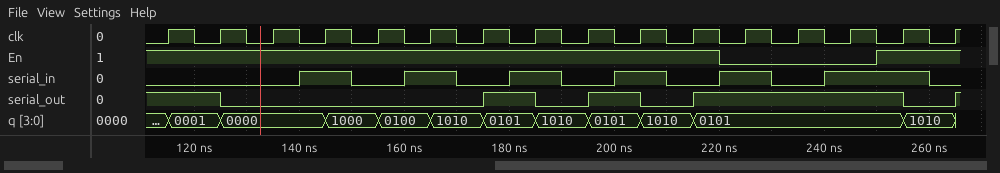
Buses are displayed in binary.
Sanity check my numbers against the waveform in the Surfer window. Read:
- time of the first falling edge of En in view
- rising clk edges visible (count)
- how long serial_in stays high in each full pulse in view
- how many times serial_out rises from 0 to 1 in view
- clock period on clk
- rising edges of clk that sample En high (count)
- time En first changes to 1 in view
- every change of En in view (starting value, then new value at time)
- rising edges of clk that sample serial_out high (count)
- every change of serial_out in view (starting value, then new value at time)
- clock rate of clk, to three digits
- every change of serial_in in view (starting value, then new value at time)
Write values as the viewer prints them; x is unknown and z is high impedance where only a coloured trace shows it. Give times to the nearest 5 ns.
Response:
220 ns
16
10 ns, 10 ns, 10 ns, 10 ns, 10 ns, 20 ns
4
10 ns
13
250 ns
1, 0 at 220 ns, 1 at 250 ns
8
1, 0 at 125 ns, 1 at 175 ns, 0 at 185 ns, 1 at 195 ns, 0 at 205 ns, 1 at 215 ns, 0 at 255 ns, 1 at 265 ns
100 MHz
0, 1 at 140 ns, 0 at 150 ns, 1 at 160 ns, 0 at 170 ns, 1 at 180 ns, 0 at 190 ns, 1 at 200 ns, 0 at 210 ns, 1 at 220 ns, 0 at 230 ns, 1 at 240 ns, 0 at 260 ns
